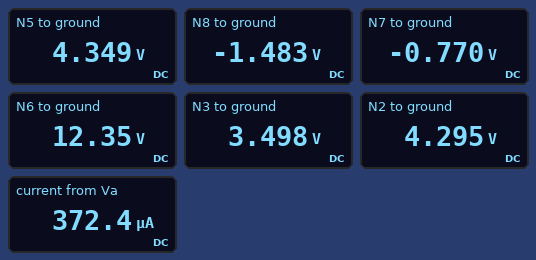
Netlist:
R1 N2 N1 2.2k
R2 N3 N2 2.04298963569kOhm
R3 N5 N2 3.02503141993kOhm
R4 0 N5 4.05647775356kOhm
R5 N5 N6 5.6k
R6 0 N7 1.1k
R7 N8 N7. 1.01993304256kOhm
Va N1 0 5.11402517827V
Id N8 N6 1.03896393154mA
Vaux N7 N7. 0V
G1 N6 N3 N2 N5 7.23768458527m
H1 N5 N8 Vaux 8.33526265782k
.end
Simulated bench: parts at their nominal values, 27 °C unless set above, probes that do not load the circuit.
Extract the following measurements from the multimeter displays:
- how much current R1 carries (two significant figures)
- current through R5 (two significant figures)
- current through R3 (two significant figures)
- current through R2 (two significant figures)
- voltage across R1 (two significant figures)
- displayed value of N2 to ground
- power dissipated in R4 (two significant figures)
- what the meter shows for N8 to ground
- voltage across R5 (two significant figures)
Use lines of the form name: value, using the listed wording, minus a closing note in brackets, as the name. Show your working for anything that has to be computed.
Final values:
how much current R1 carries: (5.114 V - 4.295 V) / 2.2 kΩ = 370 µA
current through R5: (12.35 V - 4.349 V) / 5.6 kΩ = 1.4 mA
current through R3: (4.349 V - 4.295 V) / 3.025 kΩ = 18 µA
current through R2: (4.295 V - 3.498 V) / 2.043 kΩ = 390 µA
voltage across R1: 5.114 V - 4.295 V = 820 mV
displayed value of N2 to ground: 4.295 V
power dissipated in R4: (4.349 V)^2 / 4.056 kΩ = 4.7 mW
what the meter shows for N8 to ground: -1.483 V
voltage across R5: 12.35 V - 4.349 V = 8.0 V
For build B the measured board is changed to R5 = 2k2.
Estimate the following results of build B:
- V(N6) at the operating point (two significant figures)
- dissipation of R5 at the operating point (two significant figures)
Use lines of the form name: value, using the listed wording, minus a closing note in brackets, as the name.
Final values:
V(N6) at the operating point: 7.5 V
dissipation of R5 at the operating point: 4.5 mW
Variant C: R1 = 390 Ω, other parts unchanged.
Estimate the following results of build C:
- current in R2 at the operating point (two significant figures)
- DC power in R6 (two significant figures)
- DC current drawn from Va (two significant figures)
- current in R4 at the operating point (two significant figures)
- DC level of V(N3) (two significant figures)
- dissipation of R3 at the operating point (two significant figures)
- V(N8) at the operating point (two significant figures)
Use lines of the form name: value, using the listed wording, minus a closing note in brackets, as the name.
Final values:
current in R2 at the operating point: 450 µA
DC power in R6: 710 µW
DC current drawn from Va: 430 µA
current in R4 at the operating point: 1.2 mA
DC level of V(N3): 4.0 V
dissipation of R3 at the operating point: 1.3 µW
V(N8) at the operating point: -1.7 V
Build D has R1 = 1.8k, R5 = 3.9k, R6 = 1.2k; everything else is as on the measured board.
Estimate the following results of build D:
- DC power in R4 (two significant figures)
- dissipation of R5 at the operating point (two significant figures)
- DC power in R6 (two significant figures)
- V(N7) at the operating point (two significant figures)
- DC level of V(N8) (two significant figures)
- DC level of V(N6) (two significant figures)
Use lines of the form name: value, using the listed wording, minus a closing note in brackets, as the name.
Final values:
DC power in R4: 5.0 mW
dissipation of R5 at the operating point: 8.0 mW
DC power in R6: 650 µW
V(N7) at the operating point: -880 mV
DC level of V(N8): -1.6 V
DC level of V(N6): 10 V
